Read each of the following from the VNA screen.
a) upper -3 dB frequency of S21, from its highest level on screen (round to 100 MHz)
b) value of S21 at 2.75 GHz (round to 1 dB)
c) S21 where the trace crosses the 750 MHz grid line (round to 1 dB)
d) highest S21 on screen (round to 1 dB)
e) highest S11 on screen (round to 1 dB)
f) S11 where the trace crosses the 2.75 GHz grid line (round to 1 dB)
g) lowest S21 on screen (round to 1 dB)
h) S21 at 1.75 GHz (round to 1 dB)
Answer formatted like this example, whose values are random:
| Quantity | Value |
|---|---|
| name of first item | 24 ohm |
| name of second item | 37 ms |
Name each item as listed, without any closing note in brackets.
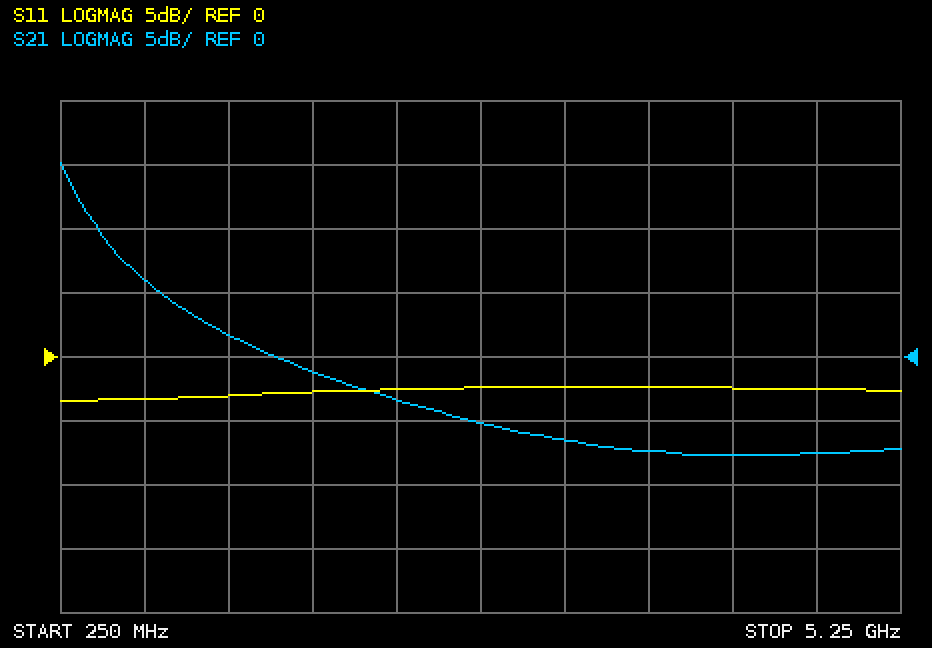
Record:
| Quantity | Value |
|---|---|
| upper -3 dB frequency of S21, from its highest level on screen | 400 MHz |
| value of S21 at 2.75 GHz | -5 dB |
| S21 where the trace crosses the 750 MHz grid line | 6 dB |
| highest S21 on screen | 15 dB |
| highest S11 on screen | -2 dB |
| S11 where the trace crosses the 2.75 GHz grid line | -2 dB |
| lowest S21 on screen | -8 dB |
| S21 at 1.75 GHz | -1 dB |
